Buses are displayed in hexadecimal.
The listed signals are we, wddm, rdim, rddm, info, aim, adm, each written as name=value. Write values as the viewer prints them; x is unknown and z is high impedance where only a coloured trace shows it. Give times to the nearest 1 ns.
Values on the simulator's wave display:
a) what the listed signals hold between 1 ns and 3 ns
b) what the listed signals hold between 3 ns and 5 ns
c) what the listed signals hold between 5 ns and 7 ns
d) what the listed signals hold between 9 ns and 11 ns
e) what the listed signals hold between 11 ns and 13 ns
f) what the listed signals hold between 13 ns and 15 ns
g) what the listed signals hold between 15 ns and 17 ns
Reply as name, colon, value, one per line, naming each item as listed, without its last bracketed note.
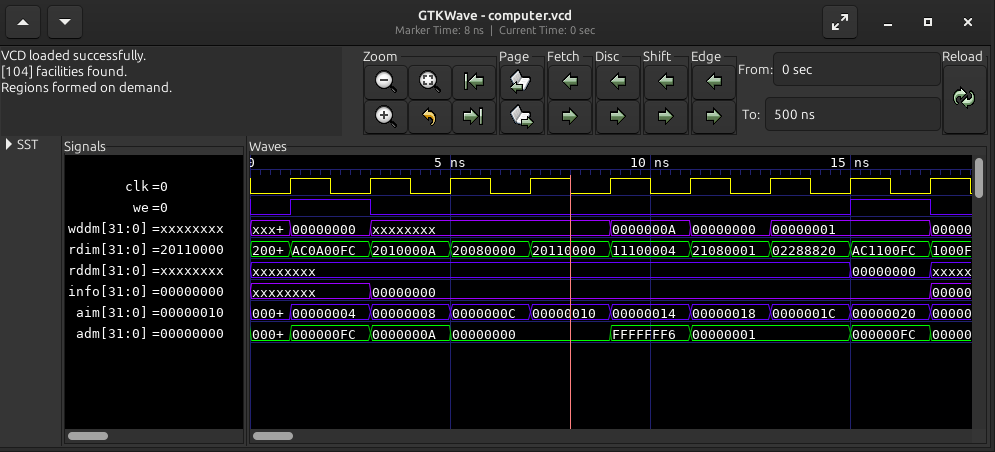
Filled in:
what the listed signals hold between 1 ns and 3 ns: we=1, wddm=00000000, rdim=AC0A00FC, rddm=xxxxxxxx, info=xxxxxxxx, aim=00000004, adm=000000FC
what the listed signals hold between 3 ns and 5 ns: we=0, wddm=xxxxxxxx, rdim=2010000A, rddm=xxxxxxxx, info=00000000, aim=00000008, adm=0000000A
what the listed signals hold between 5 ns and 7 ns: we=0, wddm=xxxxxxxx, rdim=20080000, rddm=xxxxxxxx, info=00000000, aim=0000000C, adm=00000000
what the listed signals hold between 9 ns and 11 ns: we=0, wddm=0000000A, rdim=11100004, rddm=xxxxxxxx, info=00000000, aim=00000014, adm=FFFFFFF6
what the listed signals hold between 11 ns and 13 ns: we=0, wddm=00000000, rdim=21080001, rddm=xxxxxxxx, info=00000000, aim=00000018, adm=00000001
what the listed signals hold between 13 ns and 15 ns: we=0, wddm=00000001, rdim=02288820, rddm=xxxxxxxx, info=00000000, aim=0000001C, adm=00000001
what the listed signals hold between 15 ns and 17 ns: we=1, wddm=00000001, rdim=AC1100FC, rddm=00000000, info=00000000, aim=00000020, adm=000000FC
